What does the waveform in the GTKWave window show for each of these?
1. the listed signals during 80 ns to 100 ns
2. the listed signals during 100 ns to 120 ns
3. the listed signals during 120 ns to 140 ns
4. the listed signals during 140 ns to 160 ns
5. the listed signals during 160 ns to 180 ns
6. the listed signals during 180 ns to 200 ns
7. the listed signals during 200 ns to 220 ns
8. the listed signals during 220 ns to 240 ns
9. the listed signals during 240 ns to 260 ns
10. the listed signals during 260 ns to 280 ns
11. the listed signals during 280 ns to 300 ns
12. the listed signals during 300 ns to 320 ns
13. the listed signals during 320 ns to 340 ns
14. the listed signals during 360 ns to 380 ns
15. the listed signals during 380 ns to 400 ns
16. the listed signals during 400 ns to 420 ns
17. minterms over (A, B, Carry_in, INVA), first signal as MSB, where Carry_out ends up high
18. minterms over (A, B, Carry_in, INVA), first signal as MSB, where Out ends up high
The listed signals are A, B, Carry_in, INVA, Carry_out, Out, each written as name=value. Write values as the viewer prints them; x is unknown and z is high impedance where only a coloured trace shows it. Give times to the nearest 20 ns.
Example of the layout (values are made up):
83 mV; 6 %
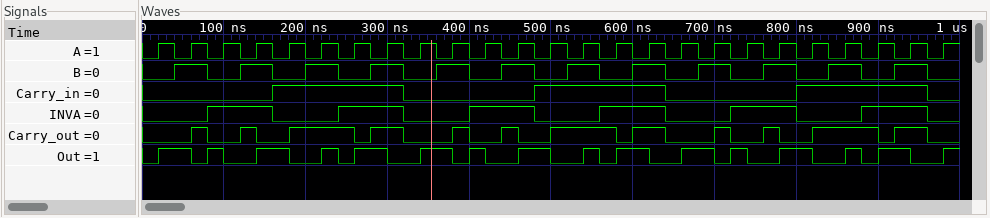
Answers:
A=0, B=0, Carry_in=0, INVA=1, Carry_out=0, Out=1; A=1, B=0, Carry_in=0, INVA=1, Carry_out=0, Out=0; A=0, B=1, Carry_in=0, INVA=1, Carry_out=1, Out=0; A=1, B=1, Carry_in=0, INVA=1, Carry_out=0, Out=1; A=0, B=0, Carry_in=1, INVA=0, Carry_out=0, Out=1; A=1, B=0, Carry_in=1, INVA=0, Carry_out=1, Out=0; A=0, B=1, Carry_in=1, INVA=0, Carry_out=1, Out=0; A=1, B=1, Carry_in=1, INVA=0, Carry_out=1, Out=1; A=0, B=0, Carry_in=1, INVA=1, Carry_out=1, Out=0; A=1, B=0, Carry_in=1, INVA=1, Carry_out=0, Out=1; A=0, B=1, Carry_in=1, INVA=1, Carry_out=1, Out=1; A=1, B=1, Carry_in=1, INVA=1, Carry_out=1, Out=0; A=0, B=0, Carry_in=0, INVA=0, Carry_out=0, Out=0; A=0, B=1, Carry_in=0, INVA=0, Carry_out=0, Out=1; A=1, B=1, Carry_in=0, INVA=0, Carry_out=1, Out=0; A=0, B=0, Carry_in=0, INVA=1, Carry_out=0, Out=1; 3, 5, 6, 7, 10, 12, 14, 15; 1, 2, 4, 7, 8, 11, 13, 14
